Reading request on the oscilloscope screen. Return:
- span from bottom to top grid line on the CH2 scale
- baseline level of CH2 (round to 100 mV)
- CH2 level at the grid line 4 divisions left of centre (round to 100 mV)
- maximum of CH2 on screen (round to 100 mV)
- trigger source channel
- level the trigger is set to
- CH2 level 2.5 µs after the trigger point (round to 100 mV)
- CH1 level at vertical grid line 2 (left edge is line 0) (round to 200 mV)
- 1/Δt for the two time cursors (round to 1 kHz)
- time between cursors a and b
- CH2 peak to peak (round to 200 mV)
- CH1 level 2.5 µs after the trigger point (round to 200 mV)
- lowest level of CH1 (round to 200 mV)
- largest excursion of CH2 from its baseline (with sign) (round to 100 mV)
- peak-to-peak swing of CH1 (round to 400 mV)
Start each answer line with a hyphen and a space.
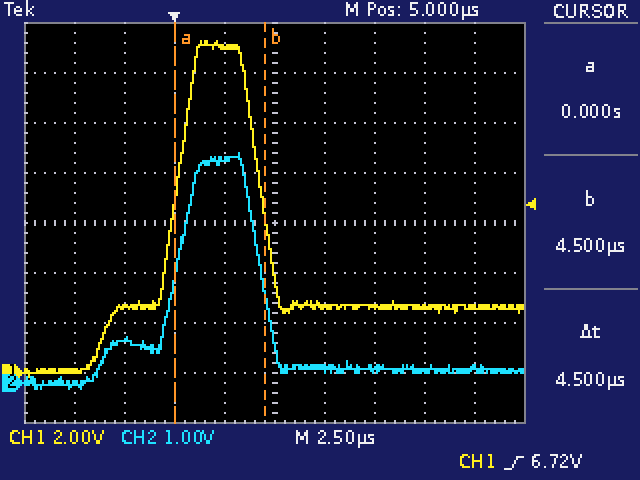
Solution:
- 8 V
- 300 mV
- 0.0 V
- 4.6 V
- CH1
- 6.72 V
- 4.5 V
- 2.6 V
- 222 kHz
- 4.5 µs
- 4.8 V
- 13.0 V
- -200 mV
- +4.3 V
- 13.6 V
